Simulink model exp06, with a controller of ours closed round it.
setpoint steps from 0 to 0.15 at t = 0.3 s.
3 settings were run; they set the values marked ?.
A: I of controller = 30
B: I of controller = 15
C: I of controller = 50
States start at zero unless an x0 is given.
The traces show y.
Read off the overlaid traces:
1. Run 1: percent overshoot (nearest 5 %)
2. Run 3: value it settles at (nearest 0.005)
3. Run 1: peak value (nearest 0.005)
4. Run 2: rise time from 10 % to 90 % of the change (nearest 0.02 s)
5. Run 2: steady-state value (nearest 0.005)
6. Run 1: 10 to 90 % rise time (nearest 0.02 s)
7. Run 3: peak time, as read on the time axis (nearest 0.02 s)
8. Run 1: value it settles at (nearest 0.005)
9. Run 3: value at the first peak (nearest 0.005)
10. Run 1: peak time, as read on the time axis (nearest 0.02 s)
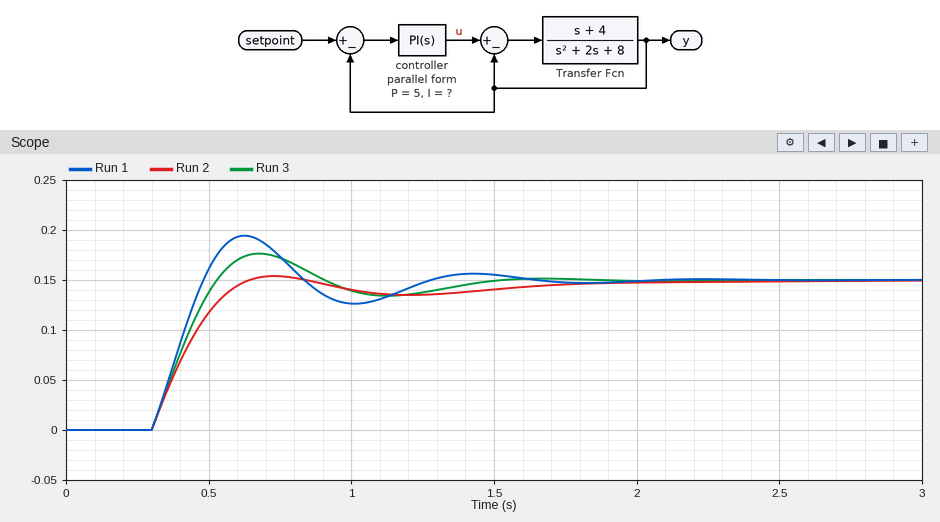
30 %
0.150
0.195
0.24 s
0.150
0.14 s
0.68 s
0.150
0.175
0.62 s
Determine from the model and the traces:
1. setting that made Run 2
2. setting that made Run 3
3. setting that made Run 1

B
A
C
